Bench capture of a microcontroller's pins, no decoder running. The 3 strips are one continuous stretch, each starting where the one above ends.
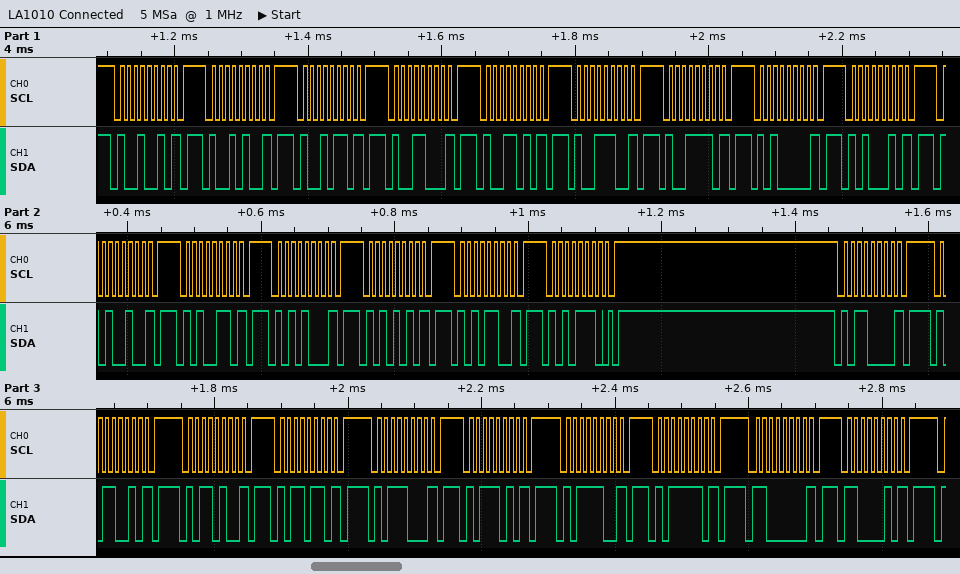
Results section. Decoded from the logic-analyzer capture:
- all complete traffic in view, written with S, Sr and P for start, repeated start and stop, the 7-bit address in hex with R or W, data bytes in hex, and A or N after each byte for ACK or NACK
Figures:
S 49W N P S 4AW N P S 4BW N P S 4CW N P S 4DW N P S 4EW N P S 4FW N P S 50W N P S 51W N P S 52W N P S 53W N P S 54W N P S 55W N P S 56W N P S 57W A P S 58W N P S 59W N P S 5AW N P S 5BW N P S 5CW N P S 5DW N P S 5EW N P S 5FW N P S 60W N P S 61W N P
